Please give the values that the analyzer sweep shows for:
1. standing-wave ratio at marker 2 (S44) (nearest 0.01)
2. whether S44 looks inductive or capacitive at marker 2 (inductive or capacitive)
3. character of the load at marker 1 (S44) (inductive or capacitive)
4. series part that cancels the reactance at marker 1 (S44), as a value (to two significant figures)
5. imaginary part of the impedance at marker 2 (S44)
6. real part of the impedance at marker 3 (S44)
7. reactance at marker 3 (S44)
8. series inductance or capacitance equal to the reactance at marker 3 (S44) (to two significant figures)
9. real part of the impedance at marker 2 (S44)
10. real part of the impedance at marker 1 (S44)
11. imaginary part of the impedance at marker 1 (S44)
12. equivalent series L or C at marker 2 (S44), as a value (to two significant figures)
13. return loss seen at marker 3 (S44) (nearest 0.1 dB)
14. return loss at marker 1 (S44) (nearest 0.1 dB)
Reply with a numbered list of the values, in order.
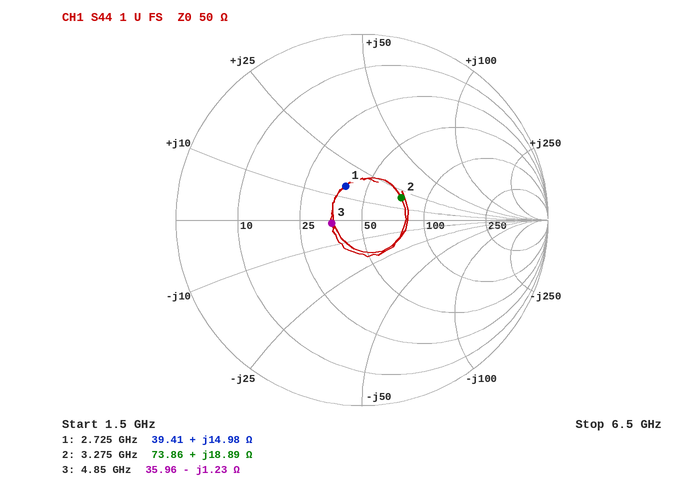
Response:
1. 1.64
2. inductive
3. inductive
4. 3.9 pF
5. +18.89 Ω
6. 35.96 Ω
7. -1.23 Ω
8. 27 pF
9. 73.86 Ω
10. 39.41 Ω
11. +14.98 Ω
12. 920 pH
13. 15.7 dB
14. 13.9 dB
